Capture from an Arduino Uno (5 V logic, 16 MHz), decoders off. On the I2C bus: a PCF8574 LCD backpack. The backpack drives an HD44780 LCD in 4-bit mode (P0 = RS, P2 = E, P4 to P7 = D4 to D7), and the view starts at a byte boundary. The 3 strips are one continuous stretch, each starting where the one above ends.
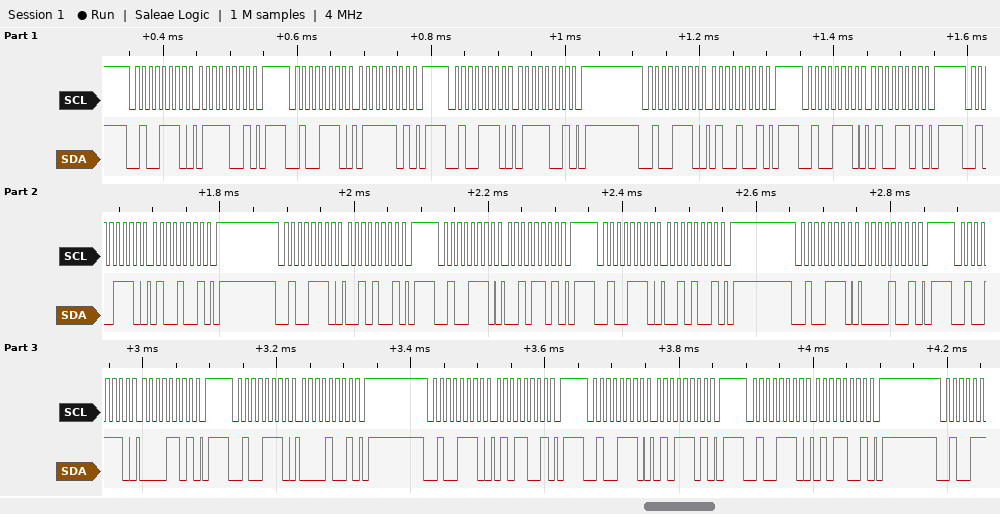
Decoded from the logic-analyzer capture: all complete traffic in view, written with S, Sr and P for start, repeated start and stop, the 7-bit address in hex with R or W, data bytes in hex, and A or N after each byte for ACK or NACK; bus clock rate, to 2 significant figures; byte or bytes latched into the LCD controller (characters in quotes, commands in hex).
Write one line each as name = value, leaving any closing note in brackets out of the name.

all complete traffic in view, written with S, Sr and P for start, repeated start and stop, the 7-bit address in hex with R or W, data bytes in hex, and A or N after each byte for ACK or NACK = S 27W A 79 A P S 27W A 7D A P S 27W A 79 A P S 27W A 49 A P S 27W A 4D A P S 27W A 49 A P S 27W A 29 A P S 27W A 2D A P S 27W A 29 A P S 27W A 09 A P S 27W A 0D A P S 27W A 09 A P S 27W A 59 A P S 27W A 5D A P S 27W A 59 A P
bus clock rate, to 2 significant figures = 100 kHz
byte or bytes latched into the LCD controller = 't' ' '
